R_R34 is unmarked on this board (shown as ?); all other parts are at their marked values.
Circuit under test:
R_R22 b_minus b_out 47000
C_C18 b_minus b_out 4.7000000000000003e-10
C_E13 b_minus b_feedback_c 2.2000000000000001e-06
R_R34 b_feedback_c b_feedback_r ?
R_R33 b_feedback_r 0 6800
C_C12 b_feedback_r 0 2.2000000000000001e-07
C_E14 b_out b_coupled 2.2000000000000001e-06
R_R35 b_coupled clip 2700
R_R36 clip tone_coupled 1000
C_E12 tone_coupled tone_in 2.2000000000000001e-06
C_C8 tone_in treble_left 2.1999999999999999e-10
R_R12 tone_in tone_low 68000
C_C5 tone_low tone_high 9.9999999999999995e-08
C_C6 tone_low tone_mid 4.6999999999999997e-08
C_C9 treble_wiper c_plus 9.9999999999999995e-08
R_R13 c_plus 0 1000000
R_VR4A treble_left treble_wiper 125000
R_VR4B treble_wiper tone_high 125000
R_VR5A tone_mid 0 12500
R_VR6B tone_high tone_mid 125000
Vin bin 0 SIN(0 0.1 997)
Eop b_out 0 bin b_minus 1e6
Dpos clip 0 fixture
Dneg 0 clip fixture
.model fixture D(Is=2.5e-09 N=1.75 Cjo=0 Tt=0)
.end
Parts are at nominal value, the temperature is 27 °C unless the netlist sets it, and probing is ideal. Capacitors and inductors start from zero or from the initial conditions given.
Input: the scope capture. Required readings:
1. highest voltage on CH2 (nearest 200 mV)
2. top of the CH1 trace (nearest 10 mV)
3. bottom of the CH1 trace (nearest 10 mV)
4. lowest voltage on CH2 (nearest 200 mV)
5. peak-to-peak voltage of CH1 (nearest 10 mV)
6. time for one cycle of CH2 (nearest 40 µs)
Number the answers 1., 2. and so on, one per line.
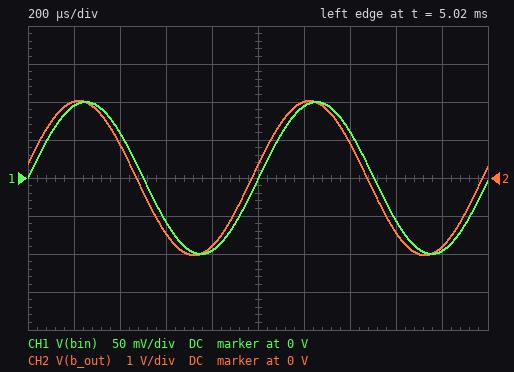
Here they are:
1. 2.0 V
2. 100 mV
3. -100 mV
4. -2.0 V
5. 200 mV
6. 1.00 ms
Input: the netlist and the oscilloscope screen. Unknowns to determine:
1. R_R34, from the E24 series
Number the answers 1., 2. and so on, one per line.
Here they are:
1. 2.2 kΩ
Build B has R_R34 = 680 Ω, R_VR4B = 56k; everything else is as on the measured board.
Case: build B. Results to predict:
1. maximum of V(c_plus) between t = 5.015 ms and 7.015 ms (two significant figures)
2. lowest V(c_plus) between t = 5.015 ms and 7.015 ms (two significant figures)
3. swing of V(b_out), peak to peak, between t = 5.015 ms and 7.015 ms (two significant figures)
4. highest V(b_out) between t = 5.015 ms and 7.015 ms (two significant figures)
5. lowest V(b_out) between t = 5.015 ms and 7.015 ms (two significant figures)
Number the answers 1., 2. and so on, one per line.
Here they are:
1. 200 mV
2. -200 mV
3. 8.7 V
4. 4.3 V
5. -4.3 V
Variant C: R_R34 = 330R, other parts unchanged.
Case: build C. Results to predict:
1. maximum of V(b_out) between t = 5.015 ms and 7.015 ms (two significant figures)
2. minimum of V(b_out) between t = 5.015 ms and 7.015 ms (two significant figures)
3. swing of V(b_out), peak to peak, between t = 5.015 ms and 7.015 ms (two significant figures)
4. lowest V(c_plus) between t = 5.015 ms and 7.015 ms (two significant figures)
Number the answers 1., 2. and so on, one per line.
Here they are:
1. 5.3 V
2. -5.3 V
3. 11 V
4. -330 mV
